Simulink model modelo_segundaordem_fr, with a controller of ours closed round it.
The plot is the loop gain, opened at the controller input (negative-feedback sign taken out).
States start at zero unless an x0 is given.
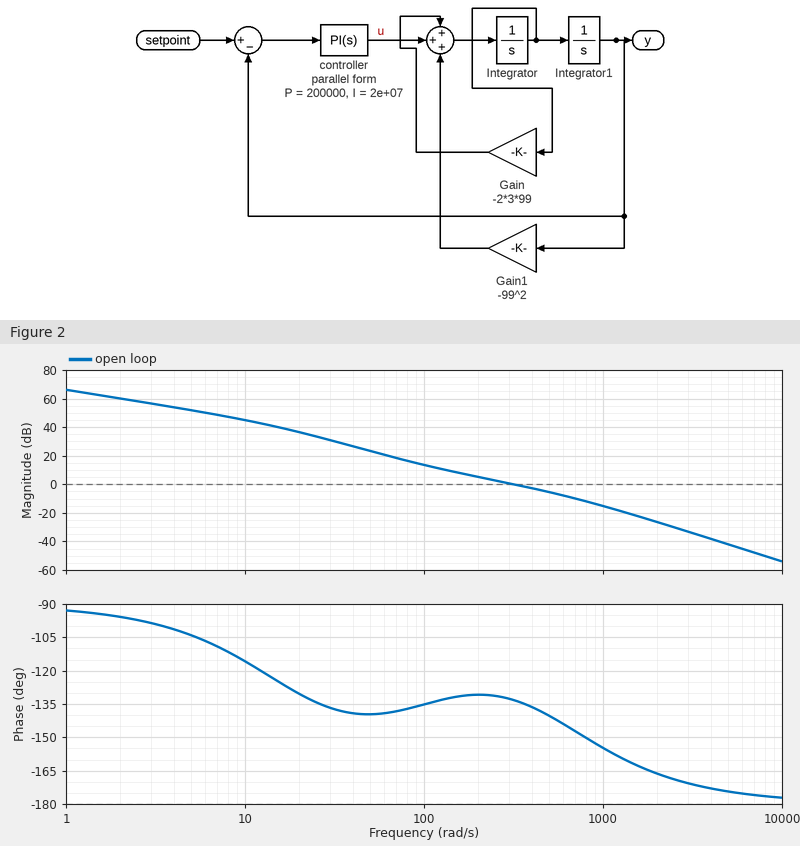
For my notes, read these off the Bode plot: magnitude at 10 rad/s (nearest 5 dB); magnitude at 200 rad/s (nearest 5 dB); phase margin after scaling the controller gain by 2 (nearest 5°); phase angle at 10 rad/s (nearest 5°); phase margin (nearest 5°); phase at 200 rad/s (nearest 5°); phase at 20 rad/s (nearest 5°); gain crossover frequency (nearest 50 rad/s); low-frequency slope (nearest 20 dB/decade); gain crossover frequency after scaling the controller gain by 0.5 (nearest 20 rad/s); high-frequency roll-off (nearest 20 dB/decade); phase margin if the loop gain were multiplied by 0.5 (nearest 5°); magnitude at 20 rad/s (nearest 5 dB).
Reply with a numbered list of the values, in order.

1. 45 dB
2. 5 dB
3. 40°
4. -115°
5. 45°
6. -130°
7. -130°
8. 300 rad/s
9. -20 dB/decade
10. 180 rad/s
11. -40 dB/decade
12. 50°
13. 35 dB
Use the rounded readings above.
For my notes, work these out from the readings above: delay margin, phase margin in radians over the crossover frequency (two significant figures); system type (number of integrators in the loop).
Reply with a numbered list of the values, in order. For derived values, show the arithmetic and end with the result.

1. 45 × π / 180 / 300 = 0.0026 s
2. 1
